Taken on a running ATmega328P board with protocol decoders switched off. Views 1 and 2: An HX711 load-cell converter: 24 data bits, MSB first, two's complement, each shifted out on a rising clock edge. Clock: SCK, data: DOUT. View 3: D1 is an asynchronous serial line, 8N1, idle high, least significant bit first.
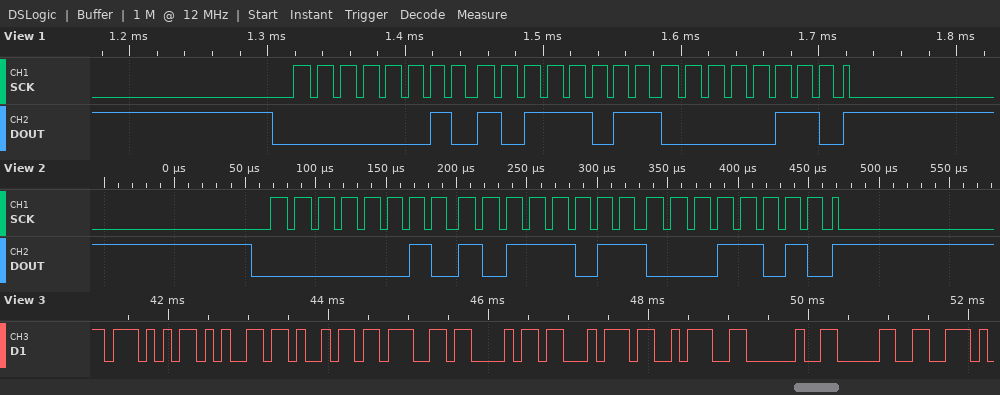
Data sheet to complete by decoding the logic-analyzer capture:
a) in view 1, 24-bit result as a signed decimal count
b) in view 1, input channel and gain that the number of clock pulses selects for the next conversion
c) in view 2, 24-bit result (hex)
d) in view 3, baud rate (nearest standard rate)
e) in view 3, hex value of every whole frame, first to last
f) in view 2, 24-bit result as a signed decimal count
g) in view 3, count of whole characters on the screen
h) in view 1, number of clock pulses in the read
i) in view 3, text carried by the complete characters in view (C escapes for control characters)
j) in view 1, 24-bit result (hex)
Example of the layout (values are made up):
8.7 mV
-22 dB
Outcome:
178950
channel A, gain 128
0x02BB1A
9600 baud
0x57 0x65 0x69 0x67 0x68 0x74 0x3A 0x20 0x30
178970
9
25
"Weight: 0"
0x02BB06
